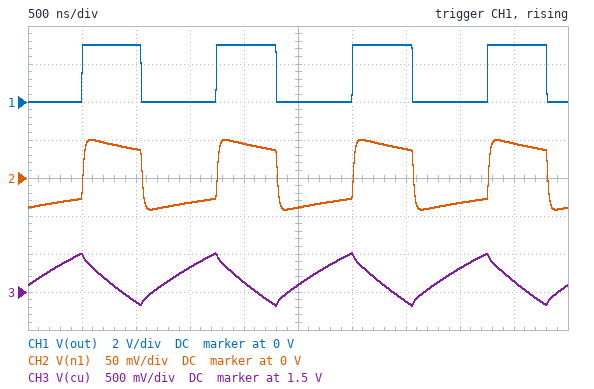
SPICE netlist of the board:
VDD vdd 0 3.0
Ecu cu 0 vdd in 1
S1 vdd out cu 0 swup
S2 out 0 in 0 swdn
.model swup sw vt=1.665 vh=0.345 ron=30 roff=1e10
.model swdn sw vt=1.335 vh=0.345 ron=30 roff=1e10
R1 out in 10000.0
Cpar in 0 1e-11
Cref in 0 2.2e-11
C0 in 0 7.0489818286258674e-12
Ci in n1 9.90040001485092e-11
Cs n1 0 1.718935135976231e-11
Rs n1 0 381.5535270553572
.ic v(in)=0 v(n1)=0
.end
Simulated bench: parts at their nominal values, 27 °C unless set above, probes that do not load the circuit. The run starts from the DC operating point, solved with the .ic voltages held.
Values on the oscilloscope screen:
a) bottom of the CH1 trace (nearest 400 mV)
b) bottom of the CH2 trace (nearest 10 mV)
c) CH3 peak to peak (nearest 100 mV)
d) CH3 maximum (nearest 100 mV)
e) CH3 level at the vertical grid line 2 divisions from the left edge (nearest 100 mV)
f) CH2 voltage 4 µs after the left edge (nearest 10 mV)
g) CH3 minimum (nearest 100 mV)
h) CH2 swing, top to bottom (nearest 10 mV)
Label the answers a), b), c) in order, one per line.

a) 0 V
b) -40 mV
c) 700 mV
d) 2.0 V
e) 1.4 V
f) -30 mV
g) 1.3 V
h) 90 mV
